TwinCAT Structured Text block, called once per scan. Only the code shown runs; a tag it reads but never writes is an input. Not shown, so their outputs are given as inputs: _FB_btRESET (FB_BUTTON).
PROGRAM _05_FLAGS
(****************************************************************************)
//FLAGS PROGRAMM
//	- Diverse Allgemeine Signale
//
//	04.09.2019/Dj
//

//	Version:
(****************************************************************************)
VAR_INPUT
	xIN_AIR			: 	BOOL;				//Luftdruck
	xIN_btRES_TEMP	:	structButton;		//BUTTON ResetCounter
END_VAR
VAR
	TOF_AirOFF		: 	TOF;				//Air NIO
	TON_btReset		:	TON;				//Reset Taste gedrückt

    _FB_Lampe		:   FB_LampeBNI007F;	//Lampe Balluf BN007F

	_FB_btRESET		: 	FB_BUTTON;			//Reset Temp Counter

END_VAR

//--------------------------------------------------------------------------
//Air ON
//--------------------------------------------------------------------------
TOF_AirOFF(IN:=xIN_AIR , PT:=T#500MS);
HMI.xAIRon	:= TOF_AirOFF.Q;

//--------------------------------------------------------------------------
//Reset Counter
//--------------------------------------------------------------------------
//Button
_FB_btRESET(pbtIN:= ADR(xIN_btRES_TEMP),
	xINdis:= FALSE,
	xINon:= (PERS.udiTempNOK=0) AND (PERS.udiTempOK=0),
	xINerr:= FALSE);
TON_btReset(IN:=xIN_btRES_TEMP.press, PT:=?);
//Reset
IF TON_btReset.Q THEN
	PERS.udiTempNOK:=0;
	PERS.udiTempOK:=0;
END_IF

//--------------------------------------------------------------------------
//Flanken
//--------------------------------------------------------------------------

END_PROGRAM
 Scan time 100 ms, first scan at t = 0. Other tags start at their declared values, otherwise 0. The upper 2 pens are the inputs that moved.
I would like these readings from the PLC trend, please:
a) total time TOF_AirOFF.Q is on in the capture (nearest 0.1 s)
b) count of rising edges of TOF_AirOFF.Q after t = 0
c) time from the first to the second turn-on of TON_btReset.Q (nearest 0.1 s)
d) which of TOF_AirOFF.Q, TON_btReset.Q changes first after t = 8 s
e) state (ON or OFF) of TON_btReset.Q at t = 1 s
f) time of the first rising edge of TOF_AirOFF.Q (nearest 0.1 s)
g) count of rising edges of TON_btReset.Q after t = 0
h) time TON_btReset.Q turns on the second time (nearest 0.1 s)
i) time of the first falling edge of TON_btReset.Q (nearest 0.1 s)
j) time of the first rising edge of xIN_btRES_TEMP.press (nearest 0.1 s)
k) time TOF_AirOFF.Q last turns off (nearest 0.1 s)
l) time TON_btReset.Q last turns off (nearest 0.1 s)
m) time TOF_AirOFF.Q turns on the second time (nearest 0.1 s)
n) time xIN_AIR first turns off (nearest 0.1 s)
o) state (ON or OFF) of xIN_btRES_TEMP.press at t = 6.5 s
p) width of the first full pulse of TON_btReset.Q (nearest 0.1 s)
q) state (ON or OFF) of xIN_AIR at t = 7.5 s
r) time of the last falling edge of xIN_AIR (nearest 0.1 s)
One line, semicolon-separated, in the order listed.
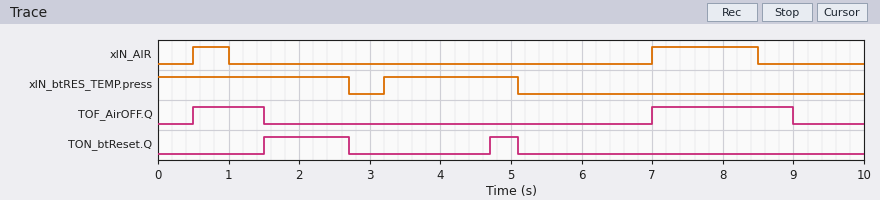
3.0 s; 2; 3.2 s; TOF_AirOFF.Q; OFF; 0.5 s; 2; 4.7 s; 2.7 s; 3.2 s; 9.0 s; 5.1 s; 7.0 s; 1.0 s; OFF; 1.2 s; ON; 8.5 s
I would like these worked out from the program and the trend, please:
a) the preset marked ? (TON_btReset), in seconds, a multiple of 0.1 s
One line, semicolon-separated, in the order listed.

1.5 s
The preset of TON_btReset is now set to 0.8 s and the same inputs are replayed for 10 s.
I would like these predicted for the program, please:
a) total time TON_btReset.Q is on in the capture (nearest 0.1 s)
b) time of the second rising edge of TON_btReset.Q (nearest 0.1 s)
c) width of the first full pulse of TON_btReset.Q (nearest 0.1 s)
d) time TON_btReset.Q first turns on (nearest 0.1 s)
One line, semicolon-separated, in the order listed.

3.0 s; 4.0 s; 1.9 s; 0.8 s
